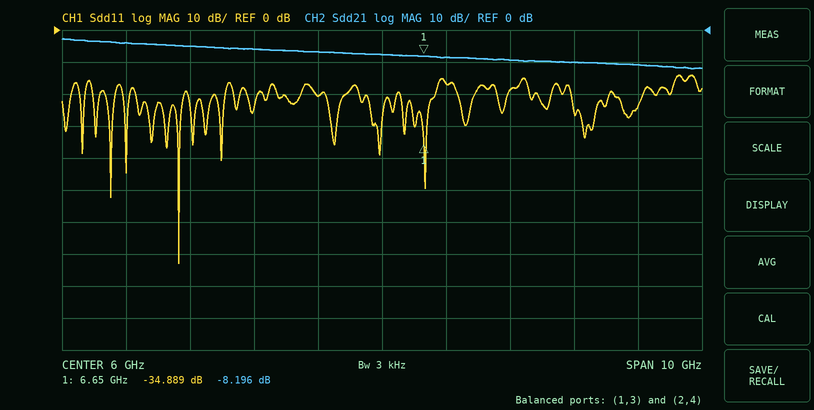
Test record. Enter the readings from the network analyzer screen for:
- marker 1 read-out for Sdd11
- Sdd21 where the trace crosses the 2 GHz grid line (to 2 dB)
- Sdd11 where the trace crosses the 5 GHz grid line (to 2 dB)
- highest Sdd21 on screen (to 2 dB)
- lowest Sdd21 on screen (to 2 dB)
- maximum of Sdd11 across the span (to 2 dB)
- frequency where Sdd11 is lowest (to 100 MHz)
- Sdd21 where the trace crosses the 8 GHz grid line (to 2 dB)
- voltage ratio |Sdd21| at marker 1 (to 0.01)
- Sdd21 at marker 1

-34.889 dB
-4 dB
-20 dB
-2 dB
-12 dB
-14 dB
2.8 GHz
-10 dB
0.39
-8.196 dB
